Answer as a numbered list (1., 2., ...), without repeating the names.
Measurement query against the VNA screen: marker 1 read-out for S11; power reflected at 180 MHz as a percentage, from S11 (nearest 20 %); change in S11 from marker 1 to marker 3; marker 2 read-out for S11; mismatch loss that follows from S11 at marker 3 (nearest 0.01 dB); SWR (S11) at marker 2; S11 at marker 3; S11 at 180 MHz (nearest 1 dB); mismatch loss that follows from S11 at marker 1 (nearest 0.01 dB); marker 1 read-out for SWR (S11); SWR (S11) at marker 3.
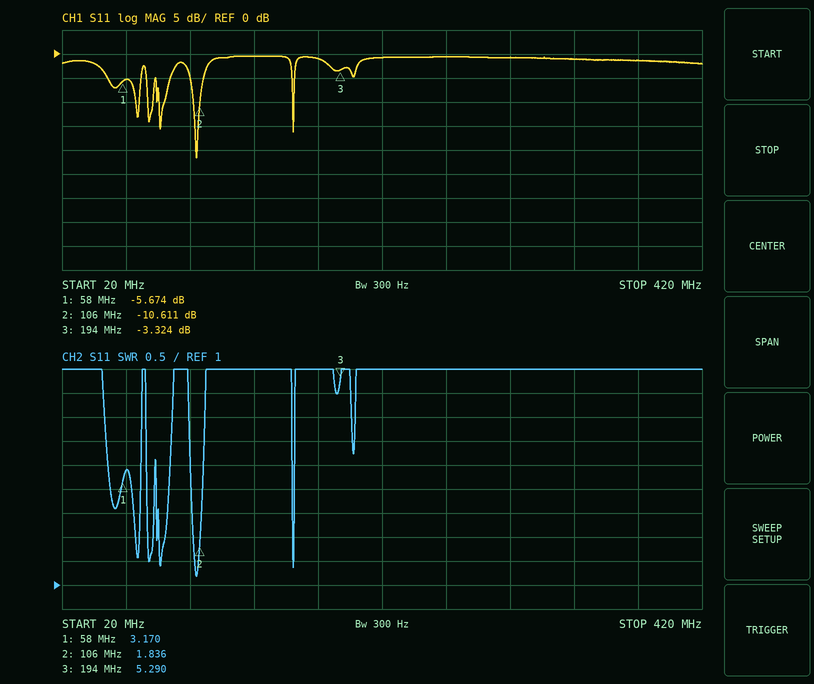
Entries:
1. -5.674 dB
2. 80 %
3. 2.350 dB
4. -10.611 dB
5. 2.72 dB
6. 1.836
7. -3.324 dB
8. -1 dB
9. 1.37 dB
10. 3.170
11. 5.290
